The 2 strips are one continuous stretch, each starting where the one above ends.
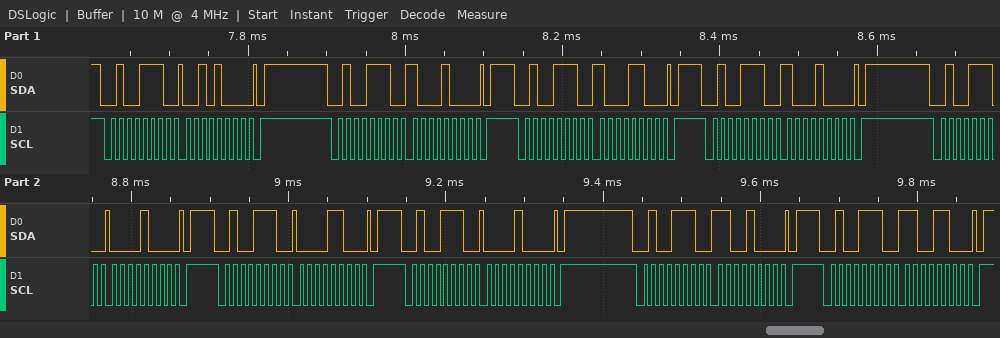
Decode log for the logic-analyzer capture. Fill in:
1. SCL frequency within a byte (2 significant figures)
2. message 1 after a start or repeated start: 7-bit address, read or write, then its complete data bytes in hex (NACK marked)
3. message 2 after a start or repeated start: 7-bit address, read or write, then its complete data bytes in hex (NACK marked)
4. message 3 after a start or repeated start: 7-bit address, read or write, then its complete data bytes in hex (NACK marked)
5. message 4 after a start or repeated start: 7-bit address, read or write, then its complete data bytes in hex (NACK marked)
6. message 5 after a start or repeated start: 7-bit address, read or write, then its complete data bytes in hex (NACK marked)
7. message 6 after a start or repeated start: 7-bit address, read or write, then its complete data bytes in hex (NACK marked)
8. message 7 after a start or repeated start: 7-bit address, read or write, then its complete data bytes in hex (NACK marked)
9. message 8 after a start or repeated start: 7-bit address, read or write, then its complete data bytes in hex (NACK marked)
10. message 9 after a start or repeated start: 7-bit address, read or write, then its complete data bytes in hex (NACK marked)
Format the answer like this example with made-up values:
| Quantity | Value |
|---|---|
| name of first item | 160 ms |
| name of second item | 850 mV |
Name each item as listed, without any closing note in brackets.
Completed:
| Quantity | Value |
|---|---|
| SCL frequency within a byte | 100 kHz |
| message 1 after a start or repeated start: 7-bit address, read or write, then its complete data bytes in hex | 0x27 write: 28 |
| message 2 after a start or repeated start: 7-bit address, read or write, then its complete data bytes in hex | 0x27 write: 88 |
| message 3 after a start or repeated start: 7-bit address, read or write, then its complete data bytes in hex | 0x27 write: 8C |
| message 4 after a start or repeated start: 7-bit address, read or write, then its complete data bytes in hex | 0x27 write: 88 |
| message 5 after a start or repeated start: 7-bit address, read or write, then its complete data bytes in hex | 0x27 write: 08 |
| message 6 after a start or repeated start: 7-bit address, read or write, then its complete data bytes in hex | 0x27 write: 0C |
| message 7 after a start or repeated start: 7-bit address, read or write, then its complete data bytes in hex | 0x27 write: 08 |
| message 8 after a start or repeated start: 7-bit address, read or write, then its complete data bytes in hex | 0x27 write: C8 |
| message 9 after a start or repeated start: 7-bit address, read or write, then its complete data bytes in hex | 0x27 write: CC |
